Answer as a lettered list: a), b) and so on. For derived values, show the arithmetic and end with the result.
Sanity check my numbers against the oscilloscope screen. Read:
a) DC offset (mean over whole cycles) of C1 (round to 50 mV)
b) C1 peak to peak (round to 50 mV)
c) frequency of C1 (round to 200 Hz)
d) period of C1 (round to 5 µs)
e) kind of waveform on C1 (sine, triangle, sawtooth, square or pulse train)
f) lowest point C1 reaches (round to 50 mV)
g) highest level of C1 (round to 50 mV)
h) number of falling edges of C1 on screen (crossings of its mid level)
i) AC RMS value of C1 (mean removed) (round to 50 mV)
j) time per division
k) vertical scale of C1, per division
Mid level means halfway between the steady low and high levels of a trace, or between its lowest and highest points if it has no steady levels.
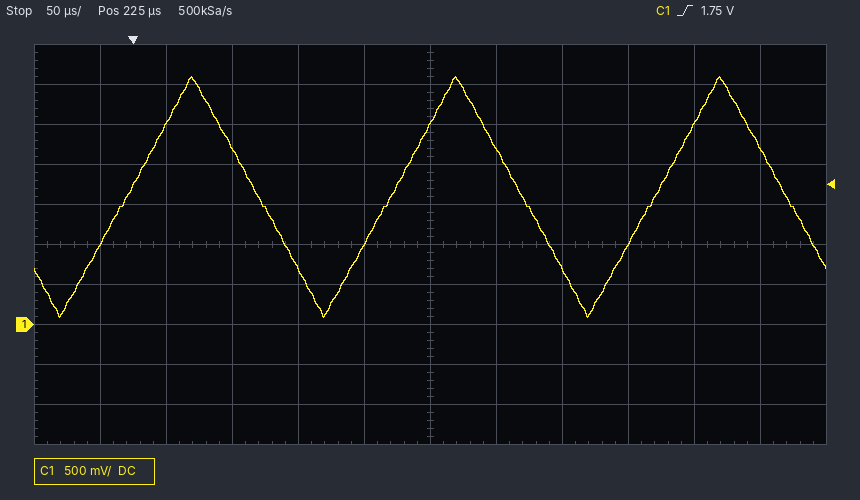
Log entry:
a) (3.10 V + (100 mV)) / 2 ≈ 1.60 V
b) 3.10 V − (100 mV) = 3.00 V
c) 1 / 200 µs ≈ 5.0 kHz
d) 200 µs
e) triangle
f) 100 mV
g) 3.10 V
h) 3
i) 3.00 V / (2√3) ≈ 866 mV, so 850 mV to the nearest 50 mV
j) 50 µs
k) 500 mV
